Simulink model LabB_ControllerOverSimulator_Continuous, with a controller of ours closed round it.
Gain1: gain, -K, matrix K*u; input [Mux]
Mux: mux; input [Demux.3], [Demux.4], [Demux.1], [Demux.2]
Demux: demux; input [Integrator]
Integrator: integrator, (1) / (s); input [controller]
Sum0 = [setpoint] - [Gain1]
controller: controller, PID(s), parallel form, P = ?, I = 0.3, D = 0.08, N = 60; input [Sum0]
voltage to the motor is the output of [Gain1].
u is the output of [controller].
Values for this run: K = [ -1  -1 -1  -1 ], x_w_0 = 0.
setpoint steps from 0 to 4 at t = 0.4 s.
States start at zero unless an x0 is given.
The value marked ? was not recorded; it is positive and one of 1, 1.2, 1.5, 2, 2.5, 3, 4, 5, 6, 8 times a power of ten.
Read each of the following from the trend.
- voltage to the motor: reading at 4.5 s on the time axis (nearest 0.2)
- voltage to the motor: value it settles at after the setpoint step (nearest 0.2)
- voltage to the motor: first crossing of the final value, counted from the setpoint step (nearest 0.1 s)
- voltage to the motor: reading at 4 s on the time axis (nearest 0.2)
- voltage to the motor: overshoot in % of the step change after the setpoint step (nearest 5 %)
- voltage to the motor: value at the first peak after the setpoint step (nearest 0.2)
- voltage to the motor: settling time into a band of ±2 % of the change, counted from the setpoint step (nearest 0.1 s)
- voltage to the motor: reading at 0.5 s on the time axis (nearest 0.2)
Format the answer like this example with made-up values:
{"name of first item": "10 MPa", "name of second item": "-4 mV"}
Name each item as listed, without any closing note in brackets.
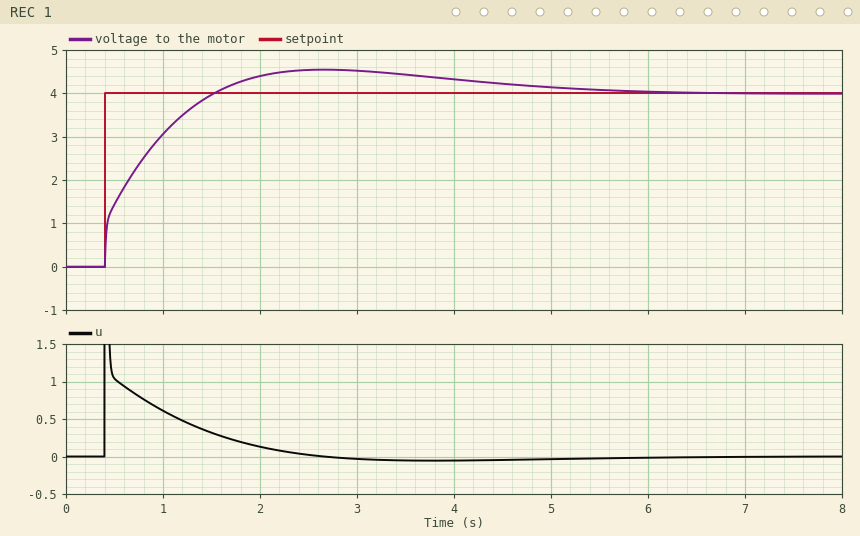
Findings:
{"voltage to the motor: reading at 4.5 s on the time axis": "4.2", "voltage to the motor: value it settles at after the setpoint step": "4.0", "voltage to the motor: first crossing of the final value, counted from the setpoint step": "1.1 s", "voltage to the motor: reading at 4 s on the time axis": "4.4", "voltage to the motor: overshoot in % of the step change after the setpoint step": "15 %", "voltage to the motor: value at the first peak after the setpoint step": "4.6", "voltage to the motor: settling time into a band of ±2 % of the change, counted from the setpoint step": "5.1 s", "voltage to the motor: reading at 0.5 s on the time axis": "1.4"}
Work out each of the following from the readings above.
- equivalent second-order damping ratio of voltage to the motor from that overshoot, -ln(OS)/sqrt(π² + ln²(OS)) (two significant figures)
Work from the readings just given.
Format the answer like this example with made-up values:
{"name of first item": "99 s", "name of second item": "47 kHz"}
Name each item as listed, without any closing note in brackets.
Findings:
{"equivalent second-order damping ratio of voltage to the motor from that overshoot, -ln(OS)/sqrt(π² + ln²(OS))": "0.52"}
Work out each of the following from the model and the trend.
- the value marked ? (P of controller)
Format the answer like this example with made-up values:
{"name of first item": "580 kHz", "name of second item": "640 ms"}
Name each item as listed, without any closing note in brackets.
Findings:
{"the value marked ?": "0.5"}
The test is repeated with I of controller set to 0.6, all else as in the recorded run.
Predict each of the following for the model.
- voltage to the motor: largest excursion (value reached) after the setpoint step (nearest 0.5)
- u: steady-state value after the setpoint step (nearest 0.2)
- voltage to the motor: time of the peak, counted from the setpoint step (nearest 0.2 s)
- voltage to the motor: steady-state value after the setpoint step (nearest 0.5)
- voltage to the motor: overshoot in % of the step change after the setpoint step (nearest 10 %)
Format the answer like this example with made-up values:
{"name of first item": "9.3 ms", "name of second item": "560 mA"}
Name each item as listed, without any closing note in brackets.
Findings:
{"voltage to the motor: largest excursion (value reached) after the setpoint step": "5.0", "u: steady-state value after the setpoint step": "0.0", "voltage to the motor: time of the peak, counted from the setpoint step": "1.8 s", "voltage to the motor: steady-state value after the setpoint step": "4.0", "voltage to the motor: overshoot in % of the step change after the setpoint step": "20 %"}
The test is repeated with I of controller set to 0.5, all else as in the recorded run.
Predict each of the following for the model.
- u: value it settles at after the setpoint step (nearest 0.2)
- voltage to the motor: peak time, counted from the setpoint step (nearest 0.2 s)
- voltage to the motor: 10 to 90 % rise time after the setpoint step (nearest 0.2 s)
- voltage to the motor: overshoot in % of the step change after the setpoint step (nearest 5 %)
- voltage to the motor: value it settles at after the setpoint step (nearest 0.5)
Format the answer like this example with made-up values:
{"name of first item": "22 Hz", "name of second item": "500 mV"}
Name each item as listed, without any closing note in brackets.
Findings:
{"u: value it settles at after the setpoint step": "0.0", "voltage to the motor: peak time, counted from the setpoint step": "1.8 s", "voltage to the motor: 10 to 90 % rise time after the setpoint step": "0.8 s", "voltage to the motor: overshoot in % of the step change after the setpoint step": "20 %", "voltage to the motor: value it settles at after the setpoint step": "4.0"}
